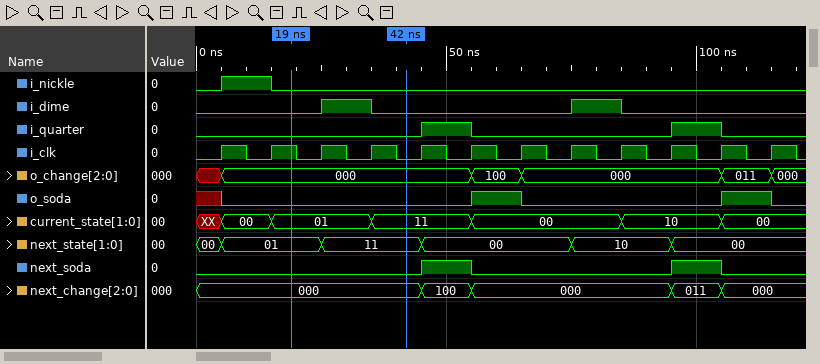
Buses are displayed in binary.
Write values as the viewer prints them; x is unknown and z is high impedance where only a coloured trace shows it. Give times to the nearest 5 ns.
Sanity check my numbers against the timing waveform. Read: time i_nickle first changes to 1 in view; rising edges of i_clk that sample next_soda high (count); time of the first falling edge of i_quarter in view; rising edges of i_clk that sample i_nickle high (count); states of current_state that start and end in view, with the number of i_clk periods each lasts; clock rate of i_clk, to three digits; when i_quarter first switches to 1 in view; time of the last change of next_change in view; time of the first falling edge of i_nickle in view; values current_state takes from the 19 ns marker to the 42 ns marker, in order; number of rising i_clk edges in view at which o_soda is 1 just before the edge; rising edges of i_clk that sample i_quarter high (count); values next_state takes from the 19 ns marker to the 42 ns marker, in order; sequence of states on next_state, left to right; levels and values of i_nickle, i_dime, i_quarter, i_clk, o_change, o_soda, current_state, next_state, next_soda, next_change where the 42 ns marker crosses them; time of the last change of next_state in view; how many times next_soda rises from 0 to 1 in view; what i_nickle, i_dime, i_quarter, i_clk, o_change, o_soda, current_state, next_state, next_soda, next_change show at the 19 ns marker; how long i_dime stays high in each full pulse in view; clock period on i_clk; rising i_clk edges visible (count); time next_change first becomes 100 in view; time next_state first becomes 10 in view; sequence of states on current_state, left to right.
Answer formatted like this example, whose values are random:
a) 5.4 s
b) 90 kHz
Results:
a) 5 ns
b) 2
c) 55 ns
d) 1
e) 00: 1, 01: 2, 11: 2, 00: 3, 10: 2
f) 100 MHz
g) 45 ns
h) 105 ns
i) 15 ns
j) 01, 11
k) 2
l) 2
m) 01, 11
n) 00, 01, 11, 00, 10, 00
o) i_nickle=0, i_dime=0, i_quarter=0, i_clk=0, o_change=000, o_soda=0, current_state=11, next_state=11, next_soda=0, next_change=000
p) 95 ns
q) 2
r) i_nickle=0, i_dime=0, i_quarter=0, i_clk=1, o_change=000, o_soda=0, current_state=01, next_state=01, next_soda=0, next_change=000
s) 10 ns, 10 ns
t) 10 ns
u) 12
v) 45 ns
w) 75 ns
x) XX, 00, 01, 11, 00, 10, 00
